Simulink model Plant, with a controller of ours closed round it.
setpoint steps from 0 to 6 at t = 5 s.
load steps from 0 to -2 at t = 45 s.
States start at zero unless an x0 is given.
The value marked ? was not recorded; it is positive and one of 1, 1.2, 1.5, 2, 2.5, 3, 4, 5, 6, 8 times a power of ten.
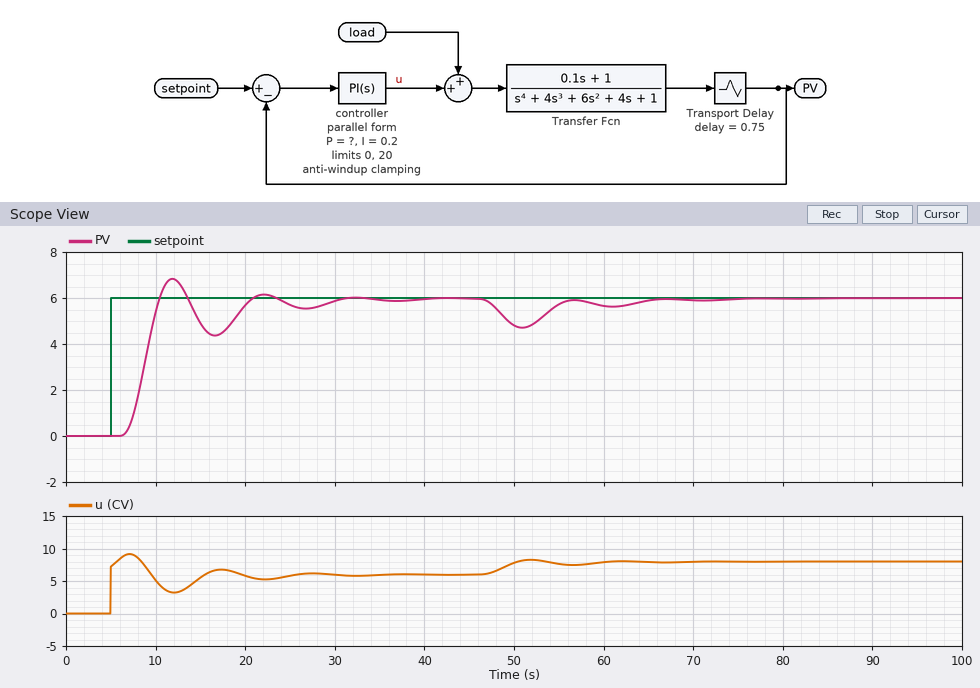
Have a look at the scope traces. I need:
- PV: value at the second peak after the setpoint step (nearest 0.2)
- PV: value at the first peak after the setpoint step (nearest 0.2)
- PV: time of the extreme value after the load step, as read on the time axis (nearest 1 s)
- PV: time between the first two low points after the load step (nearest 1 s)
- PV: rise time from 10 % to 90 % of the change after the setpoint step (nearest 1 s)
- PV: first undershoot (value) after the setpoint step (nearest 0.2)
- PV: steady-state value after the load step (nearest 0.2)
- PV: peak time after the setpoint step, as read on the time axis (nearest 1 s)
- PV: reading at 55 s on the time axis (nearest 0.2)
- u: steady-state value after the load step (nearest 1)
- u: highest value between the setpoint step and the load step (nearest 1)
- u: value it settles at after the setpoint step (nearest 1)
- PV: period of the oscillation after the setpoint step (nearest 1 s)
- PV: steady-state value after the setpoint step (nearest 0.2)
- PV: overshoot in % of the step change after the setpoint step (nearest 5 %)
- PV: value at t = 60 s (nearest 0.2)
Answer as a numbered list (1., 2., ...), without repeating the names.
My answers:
1. 6.2
2. 6.8
3. 51 s
4. 10 s
5. 3 s
6. 4.4
7. 6.0
8. 12 s
9. 5.8
10. 8
11. 9
12. 6
13. 10 s
14. 6.0
15. 15 %
16. 5.6
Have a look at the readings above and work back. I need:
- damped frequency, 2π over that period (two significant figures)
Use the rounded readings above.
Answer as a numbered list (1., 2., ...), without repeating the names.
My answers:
1. 0.63 rad/s
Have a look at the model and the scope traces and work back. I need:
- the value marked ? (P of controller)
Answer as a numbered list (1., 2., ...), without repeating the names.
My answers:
1. 1.2
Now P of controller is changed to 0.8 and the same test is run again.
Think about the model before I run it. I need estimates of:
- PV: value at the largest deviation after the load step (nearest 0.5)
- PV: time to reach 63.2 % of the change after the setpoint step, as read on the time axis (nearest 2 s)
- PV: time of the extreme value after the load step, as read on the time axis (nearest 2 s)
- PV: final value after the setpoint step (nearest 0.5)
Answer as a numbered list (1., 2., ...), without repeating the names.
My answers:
1. 4.5
2. 10 s
3. 52 s
4. 6.0
